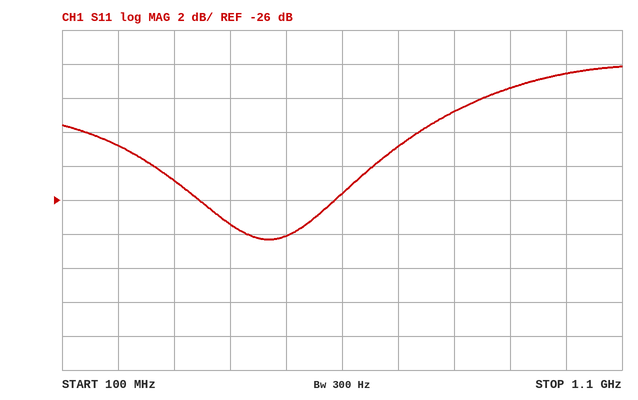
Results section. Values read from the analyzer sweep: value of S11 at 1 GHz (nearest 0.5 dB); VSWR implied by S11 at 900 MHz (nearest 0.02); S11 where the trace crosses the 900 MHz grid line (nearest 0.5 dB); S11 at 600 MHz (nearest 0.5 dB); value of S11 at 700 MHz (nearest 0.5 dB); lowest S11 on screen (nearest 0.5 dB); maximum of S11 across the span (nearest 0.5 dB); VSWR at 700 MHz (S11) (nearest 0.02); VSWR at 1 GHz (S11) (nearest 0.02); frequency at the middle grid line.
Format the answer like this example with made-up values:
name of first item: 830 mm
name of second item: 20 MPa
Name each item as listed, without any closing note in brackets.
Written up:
value of S11 at 1 GHz: -18.5 dB
VSWR implied by S11 at 900 MHz: 1.24
S11 where the trace crosses the 900 MHz grid line: -19.5 dB
S11 at 600 MHz: -25.5 dB
value of S11 at 700 MHz: -23.0 dB
lowest S11 on screen: -28.5 dB
maximum of S11 across the span: -18.0 dB
VSWR at 700 MHz (S11): 1.16
VSWR at 1 GHz (S11): 1.26
frequency at the middle grid line: 600 MHz
